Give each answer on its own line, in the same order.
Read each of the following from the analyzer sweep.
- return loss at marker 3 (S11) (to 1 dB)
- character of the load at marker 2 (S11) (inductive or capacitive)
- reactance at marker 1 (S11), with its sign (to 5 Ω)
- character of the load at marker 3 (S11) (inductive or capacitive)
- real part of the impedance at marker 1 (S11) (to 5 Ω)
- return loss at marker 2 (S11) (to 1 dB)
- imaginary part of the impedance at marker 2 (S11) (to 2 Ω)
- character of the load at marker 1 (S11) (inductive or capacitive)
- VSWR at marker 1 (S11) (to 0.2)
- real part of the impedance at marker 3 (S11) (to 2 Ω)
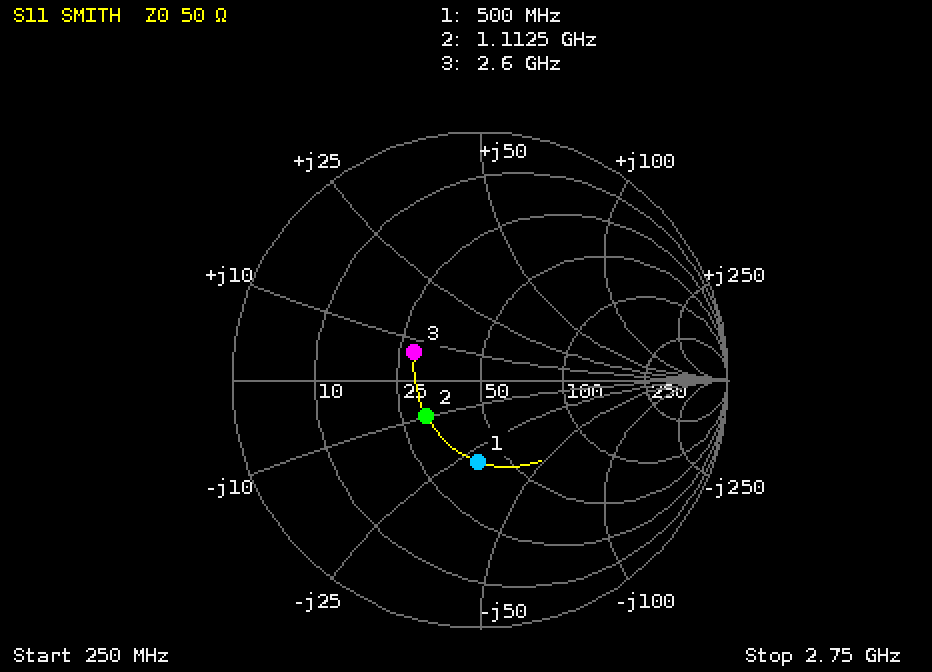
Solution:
11 dB
capacitive
-30 Ω
inductive
40 Ω
12 dB
-10 Ω
capacitive
2.0
28 Ω
